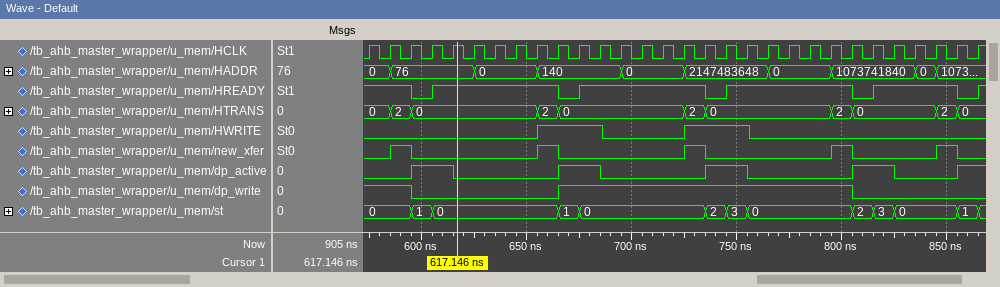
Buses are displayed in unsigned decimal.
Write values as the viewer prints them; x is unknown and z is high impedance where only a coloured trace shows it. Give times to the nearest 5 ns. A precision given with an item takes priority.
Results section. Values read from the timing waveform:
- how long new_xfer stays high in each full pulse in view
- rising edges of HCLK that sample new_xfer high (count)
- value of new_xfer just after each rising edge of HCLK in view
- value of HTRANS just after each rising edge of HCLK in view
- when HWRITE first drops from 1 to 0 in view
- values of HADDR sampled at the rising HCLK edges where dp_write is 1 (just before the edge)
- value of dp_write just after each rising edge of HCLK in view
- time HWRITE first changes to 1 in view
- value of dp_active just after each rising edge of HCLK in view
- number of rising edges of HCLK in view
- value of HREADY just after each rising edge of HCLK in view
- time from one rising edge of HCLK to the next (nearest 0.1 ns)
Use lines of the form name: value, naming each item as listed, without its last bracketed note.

how long new_xfer stays high in each full pulse in view: 10 ns, 10 ns, 10 ns, 10 ns, 10 ns
rising edges of HCLK that sample new_xfer high: 5
value of new_xfer just after each rising edge of HCLK in view: 0 1 0 0 0 0 0 0 1 0 0 0 0 0 0 1 0 0 0 0 0 0 1 0 0 0 0 1 0 0
value of HTRANS just after each rising edge of HCLK in view: 0, 2, 0, 0, 0, 0, 0, 0, 2, 0, 0, 0, 0, 0, 0, 2, 0, 0, 0, 0, 0, 0, 2, 0, 0, 0, 0, 2, 0, 0
when HWRITE first drops from 1 to 0 in view: 685 ns
values of HADDR sampled at the rising HCLK edges where dp_write is 1: 0, 0, 76, 140, 140, 140, 0, 0, 0, 2147483648, 2147483648, 2147483648, 2147483648, 0, 0, 0, 1073741840
value of dp_write just after each rising edge of HCLK in view: 1 1 0 0 0 0 0 0 0 1 1 1 1 1 1 1 1 1 1 1 1 1 1 0 0 0 0 0 0 0
time HWRITE first changes to 1 in view: 655 ns
value of dp_active just after each rising edge of HCLK in view: 0 0 1 1 0 0 0 0 0 1 1 0 0 0 0 0 1 1 0 0 0 0 0 1 1 0 0 0 1 1
number of rising edges of HCLK in view: 30
value of HREADY just after each rising edge of HCLK in view: 1 1 0 1 1 1 1 1 1 0 1 1 1 1 1 1 0 1 1 1 1 1 1 0 1 1 1 1 0 1
time from one rising edge of HCLK to the next: 10 ns
